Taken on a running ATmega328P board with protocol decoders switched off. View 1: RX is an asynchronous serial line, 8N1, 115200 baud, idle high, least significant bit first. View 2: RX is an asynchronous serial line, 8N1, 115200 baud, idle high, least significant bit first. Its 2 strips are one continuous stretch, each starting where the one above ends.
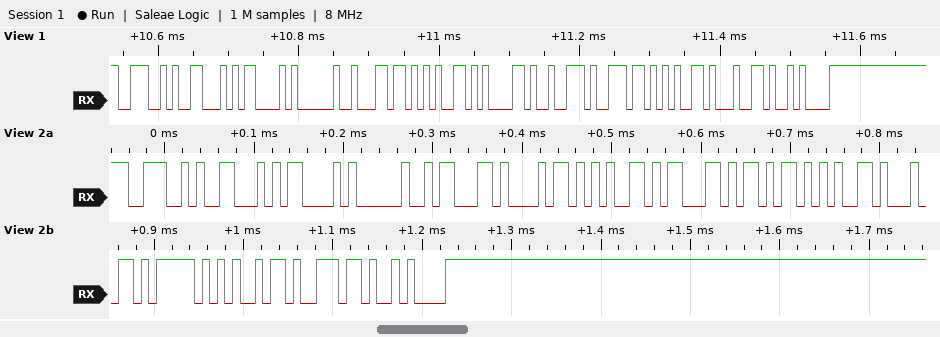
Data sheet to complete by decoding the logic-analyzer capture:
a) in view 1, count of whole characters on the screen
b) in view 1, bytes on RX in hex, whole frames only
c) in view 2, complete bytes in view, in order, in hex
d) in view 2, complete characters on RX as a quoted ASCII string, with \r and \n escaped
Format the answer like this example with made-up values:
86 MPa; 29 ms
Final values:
12; 0x4E 0x46 0x43 0x20 0x6C 0x65 0x61 0x72 0x6E 0x65 0x64 0x0A; 4E 46 43 20 63 68 65 63 6B 65 64 5F 69 6E 0A; "NFC checked_in\n"
